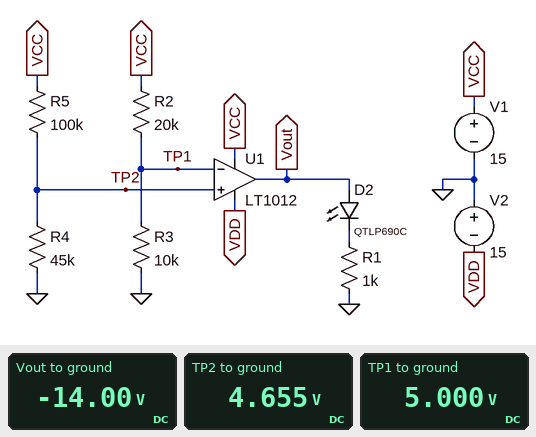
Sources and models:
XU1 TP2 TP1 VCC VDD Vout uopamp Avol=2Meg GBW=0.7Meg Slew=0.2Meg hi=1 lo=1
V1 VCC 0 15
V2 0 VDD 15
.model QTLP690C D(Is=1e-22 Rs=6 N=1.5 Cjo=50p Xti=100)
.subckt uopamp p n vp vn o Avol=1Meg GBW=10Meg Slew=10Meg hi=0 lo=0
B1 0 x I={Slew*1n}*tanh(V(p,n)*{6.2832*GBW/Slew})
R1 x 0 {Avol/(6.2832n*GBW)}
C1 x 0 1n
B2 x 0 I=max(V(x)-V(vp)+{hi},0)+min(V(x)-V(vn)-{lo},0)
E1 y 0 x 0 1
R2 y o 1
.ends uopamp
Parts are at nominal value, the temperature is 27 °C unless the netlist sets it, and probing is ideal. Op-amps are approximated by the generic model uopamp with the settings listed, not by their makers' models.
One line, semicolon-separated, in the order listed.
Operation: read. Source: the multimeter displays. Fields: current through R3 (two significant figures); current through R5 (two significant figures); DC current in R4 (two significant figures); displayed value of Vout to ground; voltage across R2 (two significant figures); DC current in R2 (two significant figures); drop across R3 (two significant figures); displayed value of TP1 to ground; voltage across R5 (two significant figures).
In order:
500 µA; 100 µA; 100 µA; -14.00 V; 10 V; 500 µA; 5.0 V; 5.000 V; 10 V
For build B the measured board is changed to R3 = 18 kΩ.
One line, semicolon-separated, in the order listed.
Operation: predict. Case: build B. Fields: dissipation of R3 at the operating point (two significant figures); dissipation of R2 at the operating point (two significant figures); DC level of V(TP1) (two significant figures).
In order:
2.8 mW; 3.1 mW; 7.1 V
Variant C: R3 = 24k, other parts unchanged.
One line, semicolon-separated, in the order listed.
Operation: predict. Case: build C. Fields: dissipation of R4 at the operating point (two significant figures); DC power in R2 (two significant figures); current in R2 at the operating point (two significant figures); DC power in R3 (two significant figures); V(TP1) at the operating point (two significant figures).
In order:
480 µW; 2.3 mW; 340 µA; 2.8 mW; 8.2 V
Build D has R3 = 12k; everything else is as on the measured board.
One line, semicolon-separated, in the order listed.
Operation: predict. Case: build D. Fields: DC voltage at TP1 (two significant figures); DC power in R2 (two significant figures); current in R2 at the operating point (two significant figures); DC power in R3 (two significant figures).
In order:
5.6 V; 4.4 mW; 470 µA; 2.6 mW
